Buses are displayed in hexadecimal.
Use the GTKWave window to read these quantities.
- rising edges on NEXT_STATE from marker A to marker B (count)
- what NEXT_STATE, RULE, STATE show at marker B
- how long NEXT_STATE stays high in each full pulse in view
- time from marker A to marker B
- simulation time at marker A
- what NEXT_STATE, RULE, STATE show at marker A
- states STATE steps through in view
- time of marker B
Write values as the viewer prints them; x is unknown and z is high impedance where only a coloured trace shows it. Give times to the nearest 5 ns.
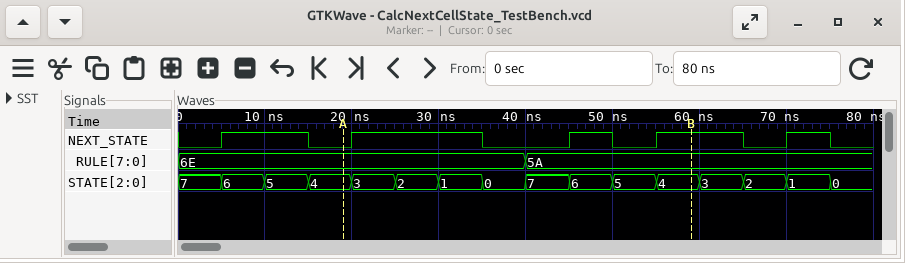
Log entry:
3
NEXT_STATE=1, RULE=5A, STATE=4
10 ns, 15 ns, 5 ns, 10 ns, 5 ns
40 ns
20 ns
NEXT_STATE=0, RULE=6E, STATE=4
7, 6, 5, 4, 3, 2, 1, 0, 7, 6, 5, 4, 3, 2, 1, 0
60 ns
